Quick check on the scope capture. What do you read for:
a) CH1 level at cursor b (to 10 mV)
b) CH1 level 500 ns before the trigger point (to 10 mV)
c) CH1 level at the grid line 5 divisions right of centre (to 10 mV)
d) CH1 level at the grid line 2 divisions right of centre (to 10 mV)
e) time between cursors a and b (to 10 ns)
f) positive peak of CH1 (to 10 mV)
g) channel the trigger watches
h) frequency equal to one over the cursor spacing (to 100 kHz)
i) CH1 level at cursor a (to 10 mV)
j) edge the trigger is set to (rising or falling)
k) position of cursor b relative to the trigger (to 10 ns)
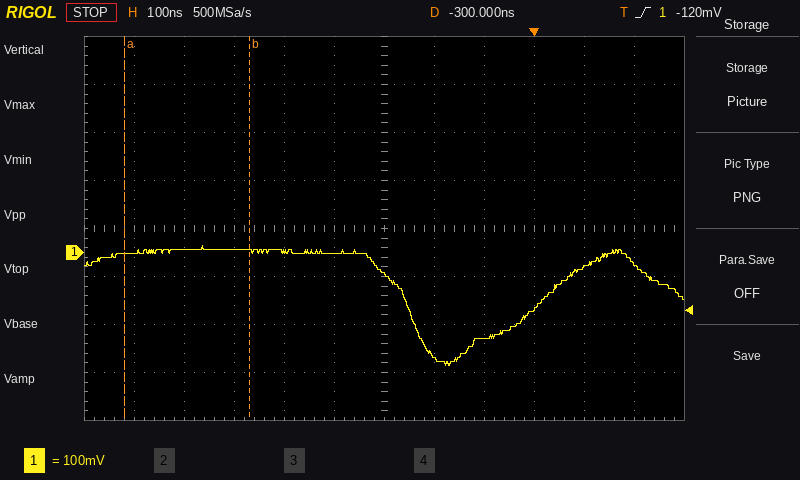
0 mV
0 mV
-20 mV
-180 mV
250 ns
10 mV
CH1
4.0 MHz
0 mV
rising
-570 ns
